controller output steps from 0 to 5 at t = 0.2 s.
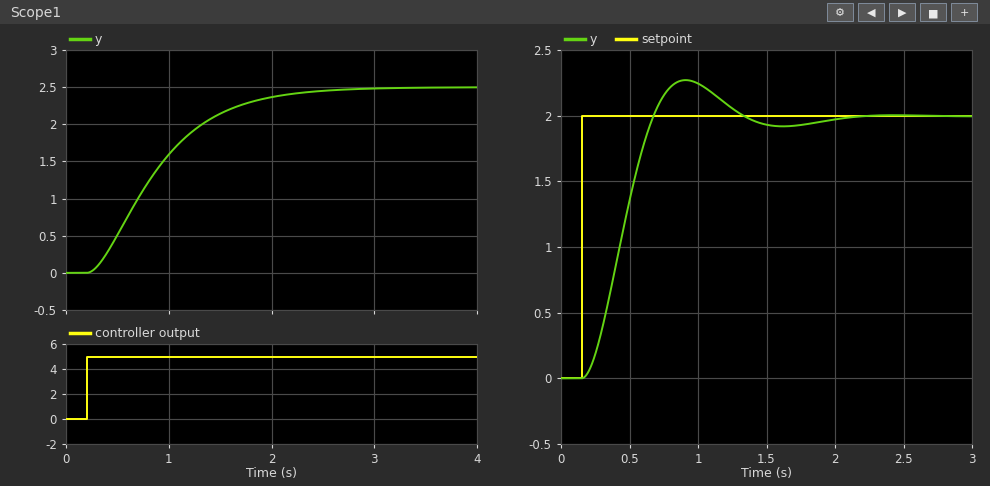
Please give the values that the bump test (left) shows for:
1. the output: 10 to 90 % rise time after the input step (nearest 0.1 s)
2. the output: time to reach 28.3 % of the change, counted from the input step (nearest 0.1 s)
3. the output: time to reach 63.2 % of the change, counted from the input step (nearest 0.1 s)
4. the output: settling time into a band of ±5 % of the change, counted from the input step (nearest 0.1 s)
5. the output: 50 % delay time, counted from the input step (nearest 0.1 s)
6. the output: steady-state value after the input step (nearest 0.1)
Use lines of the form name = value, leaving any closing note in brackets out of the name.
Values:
the output: 10 to 90 % rise time after the input step = 1.3 s
the output: time to reach 28.3 % of the change, counted from the input step = 0.4 s
the output: time to reach 63.2 % of the change, counted from the input step = 0.8 s
the output: settling time into a band of ±5 % of the change, counted from the input step = 1.8 s
the output: 50 % delay time, counted from the input step = 0.6 s
the output: steady-state value after the input step = 2.5
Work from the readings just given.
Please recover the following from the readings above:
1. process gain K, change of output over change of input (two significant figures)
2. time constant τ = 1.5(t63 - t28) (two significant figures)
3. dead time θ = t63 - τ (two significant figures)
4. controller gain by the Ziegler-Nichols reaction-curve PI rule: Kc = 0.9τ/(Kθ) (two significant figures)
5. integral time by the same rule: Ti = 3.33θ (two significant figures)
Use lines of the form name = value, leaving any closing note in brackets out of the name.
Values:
process gain K, change of output over change of input = 0.50
time constant τ = 1.5(t63 - t28) = 0.60 s
dead time θ = t63 - τ = 0.20 s
controller gain by the Ziegler-Nichols reaction-curve PI rule: Kc = 0.9τ/(Kθ) = 5.4
integral time by the same rule: Ti = 3.33θ = 0.67 s
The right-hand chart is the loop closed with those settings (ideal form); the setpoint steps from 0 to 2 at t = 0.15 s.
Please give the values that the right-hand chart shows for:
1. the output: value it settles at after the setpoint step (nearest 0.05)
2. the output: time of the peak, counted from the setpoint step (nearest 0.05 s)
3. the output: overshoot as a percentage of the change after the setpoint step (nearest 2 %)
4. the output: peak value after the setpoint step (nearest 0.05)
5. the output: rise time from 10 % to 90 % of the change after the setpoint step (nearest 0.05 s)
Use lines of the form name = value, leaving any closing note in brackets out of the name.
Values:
the output: value it settles at after the setpoint step = 2.00
the output: time of the peak, counted from the setpoint step = 0.75 s
the output: overshoot as a percentage of the change after the setpoint step = 14 %
the output: peak value after the setpoint step = 2.25
the output: rise time from 10 % to 90 % of the change after the setpoint step = 0.35 s
